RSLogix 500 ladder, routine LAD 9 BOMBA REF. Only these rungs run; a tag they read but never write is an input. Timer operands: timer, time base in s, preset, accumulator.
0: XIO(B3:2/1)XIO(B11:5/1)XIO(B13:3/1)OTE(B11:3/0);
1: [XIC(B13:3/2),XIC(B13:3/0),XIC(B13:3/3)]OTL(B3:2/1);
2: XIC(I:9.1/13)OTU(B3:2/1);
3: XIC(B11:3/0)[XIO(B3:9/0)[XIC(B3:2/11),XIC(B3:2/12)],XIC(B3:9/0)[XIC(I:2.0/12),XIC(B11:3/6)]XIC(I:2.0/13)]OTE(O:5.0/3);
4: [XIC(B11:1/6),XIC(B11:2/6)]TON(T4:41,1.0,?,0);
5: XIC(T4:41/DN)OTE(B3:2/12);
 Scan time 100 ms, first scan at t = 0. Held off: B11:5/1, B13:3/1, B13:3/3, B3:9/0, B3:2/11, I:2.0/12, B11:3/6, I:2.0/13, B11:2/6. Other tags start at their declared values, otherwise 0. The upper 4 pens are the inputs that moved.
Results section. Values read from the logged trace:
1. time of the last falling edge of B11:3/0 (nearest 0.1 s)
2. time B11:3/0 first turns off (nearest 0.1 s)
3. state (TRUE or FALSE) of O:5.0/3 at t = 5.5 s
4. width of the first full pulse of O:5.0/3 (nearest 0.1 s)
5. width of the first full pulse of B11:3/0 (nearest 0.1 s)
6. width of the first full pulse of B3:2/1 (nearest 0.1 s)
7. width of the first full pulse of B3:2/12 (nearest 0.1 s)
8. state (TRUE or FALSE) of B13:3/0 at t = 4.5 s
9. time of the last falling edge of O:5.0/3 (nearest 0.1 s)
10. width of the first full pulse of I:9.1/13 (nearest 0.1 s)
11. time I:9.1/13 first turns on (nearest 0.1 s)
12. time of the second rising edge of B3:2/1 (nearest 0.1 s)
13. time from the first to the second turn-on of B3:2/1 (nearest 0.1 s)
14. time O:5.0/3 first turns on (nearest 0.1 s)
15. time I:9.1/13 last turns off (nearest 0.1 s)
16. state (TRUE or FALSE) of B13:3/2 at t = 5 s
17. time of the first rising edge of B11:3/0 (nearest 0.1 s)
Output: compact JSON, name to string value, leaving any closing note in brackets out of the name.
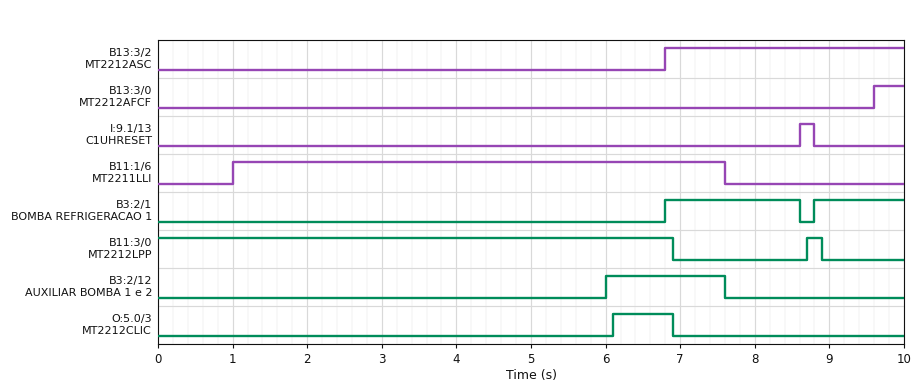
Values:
{"time of the last falling edge of B11:3/0": "8.9 s", "time B11:3/0 first turns off": "6.9 s", "state (TRUE or FALSE) of O:5.0/3 at t = 5.5 s": "FALSE", "width of the first full pulse of O:5.0/3": "0.8 s", "width of the first full pulse of B11:3/0": "0.2 s", "width of the first full pulse of B3:2/1": "1.8 s", "width of the first full pulse of B3:2/12": "1.6 s", "state (TRUE or FALSE) of B13:3/0 at t = 4.5 s": "FALSE", "time of the last falling edge of O:5.0/3": "6.9 s", "width of the first full pulse of I:9.1/13": "0.2 s", "time I:9.1/13 first turns on": "8.6 s", "time of the second rising edge of B3:2/1": "8.8 s", "time from the first to the second turn-on of B3:2/1": "2.0 s", "time O:5.0/3 first turns on": "6.1 s", "time I:9.1/13 last turns off": "8.8 s", "state (TRUE or FALSE) of B13:3/2 at t = 5 s": "FALSE", "time of the first rising edge of B11:3/0": "8.7 s"}
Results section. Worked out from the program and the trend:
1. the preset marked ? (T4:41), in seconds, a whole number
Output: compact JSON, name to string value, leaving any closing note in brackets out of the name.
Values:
{"the preset marked ? (T4:41), in seconds, a whole number": "5 s"}
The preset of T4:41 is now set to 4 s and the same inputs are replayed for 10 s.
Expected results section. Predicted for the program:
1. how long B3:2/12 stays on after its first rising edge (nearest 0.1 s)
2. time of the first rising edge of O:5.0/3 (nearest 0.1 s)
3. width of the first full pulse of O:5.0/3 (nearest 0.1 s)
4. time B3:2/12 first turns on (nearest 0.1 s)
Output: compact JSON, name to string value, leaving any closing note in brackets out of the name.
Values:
{"how long B3:2/12 stays on after its first rising edge": "2.6 s", "time of the first rising edge of O:5.0/3": "5.1 s", "width of the first full pulse of O:5.0/3": "1.8 s", "time B3:2/12 first turns on": "5.0 s"}
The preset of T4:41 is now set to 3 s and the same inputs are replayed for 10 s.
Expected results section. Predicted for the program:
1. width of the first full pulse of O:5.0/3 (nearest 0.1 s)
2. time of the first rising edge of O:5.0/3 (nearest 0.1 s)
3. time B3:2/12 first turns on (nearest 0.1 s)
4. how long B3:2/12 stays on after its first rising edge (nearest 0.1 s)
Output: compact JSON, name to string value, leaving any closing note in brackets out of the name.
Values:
{"width of the first full pulse of O:5.0/3": "2.8 s", "time of the first rising edge of O:5.0/3": "4.1 s", "time B3:2/12 first turns on": "4.0 s", "how long B3:2/12 stays on after its first rising edge": "3.6 s"}
